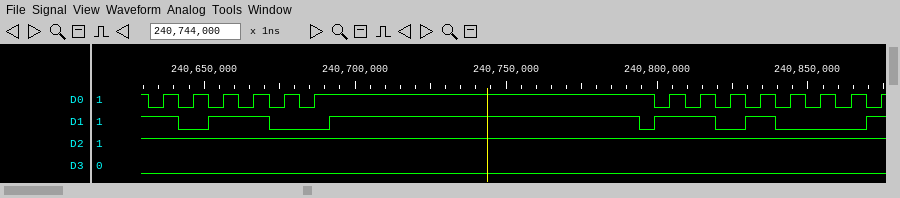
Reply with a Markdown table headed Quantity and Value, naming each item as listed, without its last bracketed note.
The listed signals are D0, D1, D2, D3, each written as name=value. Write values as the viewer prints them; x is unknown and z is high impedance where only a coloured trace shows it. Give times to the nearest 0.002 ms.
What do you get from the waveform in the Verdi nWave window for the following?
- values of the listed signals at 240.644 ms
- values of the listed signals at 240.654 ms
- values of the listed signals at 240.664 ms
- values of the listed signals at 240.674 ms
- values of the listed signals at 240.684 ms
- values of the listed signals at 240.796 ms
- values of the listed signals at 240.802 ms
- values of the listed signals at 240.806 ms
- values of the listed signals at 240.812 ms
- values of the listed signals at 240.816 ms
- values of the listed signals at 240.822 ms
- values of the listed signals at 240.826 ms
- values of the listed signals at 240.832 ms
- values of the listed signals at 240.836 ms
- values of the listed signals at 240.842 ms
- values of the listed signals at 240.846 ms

| Quantity | Value |
|---|---|
| values of the listed signals at 240.644 ms | D0=0, D1=0, D2=1, D3=0 |
| values of the listed signals at 240.654 ms | D0=0, D1=1, D2=1, D3=0 |
| values of the listed signals at 240.664 ms | D0=0, D1=1, D2=1, D3=0 |
| values of the listed signals at 240.674 ms | D0=0, D1=0, D2=1, D3=0 |
| values of the listed signals at 240.684 ms | D0=0, D1=0, D2=1, D3=0 |
| values of the listed signals at 240.796 ms | D0=1, D1=0, D2=1, D3=0 |
| values of the listed signals at 240.802 ms | D0=0, D1=1, D2=1, D3=0 |
| values of the listed signals at 240.806 ms | D0=1, D1=1, D2=1, D3=0 |
| values of the listed signals at 240.812 ms | D0=0, D1=1, D2=1, D3=0 |
| values of the listed signals at 240.816 ms | D0=1, D1=1, D2=1, D3=0 |
| values of the listed signals at 240.822 ms | D0=0, D1=0, D2=1, D3=0 |
| values of the listed signals at 240.826 ms | D0=1, D1=0, D2=1, D3=0 |
| values of the listed signals at 240.832 ms | D0=0, D1=1, D2=1, D3=0 |
| values of the listed signals at 240.836 ms | D0=1, D1=1, D2=1, D3=0 |
| values of the listed signals at 240.842 ms | D0=0, D1=0, D2=1, D3=0 |
| values of the listed signals at 240.846 ms | D0=1, D1=0, D2=1, D3=0 |
